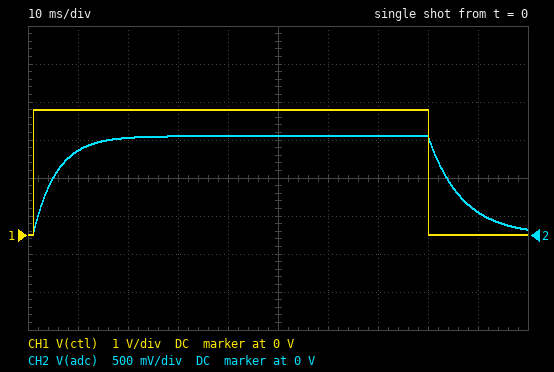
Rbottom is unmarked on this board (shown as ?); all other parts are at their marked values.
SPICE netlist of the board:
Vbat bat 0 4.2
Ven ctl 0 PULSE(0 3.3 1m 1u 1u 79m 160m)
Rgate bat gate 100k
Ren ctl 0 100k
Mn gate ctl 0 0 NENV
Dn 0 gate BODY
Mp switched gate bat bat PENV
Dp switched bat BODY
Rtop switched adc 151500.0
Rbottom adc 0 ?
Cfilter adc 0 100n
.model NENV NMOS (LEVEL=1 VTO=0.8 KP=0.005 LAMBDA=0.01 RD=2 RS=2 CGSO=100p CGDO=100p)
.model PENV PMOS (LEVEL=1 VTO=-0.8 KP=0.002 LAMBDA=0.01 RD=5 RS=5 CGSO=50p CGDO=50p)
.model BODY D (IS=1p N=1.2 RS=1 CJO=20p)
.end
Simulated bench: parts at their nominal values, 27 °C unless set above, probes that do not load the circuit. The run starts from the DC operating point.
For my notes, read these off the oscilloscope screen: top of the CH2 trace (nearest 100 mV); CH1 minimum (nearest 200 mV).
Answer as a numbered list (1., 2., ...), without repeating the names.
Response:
1. 1.3 V
2. 0 V
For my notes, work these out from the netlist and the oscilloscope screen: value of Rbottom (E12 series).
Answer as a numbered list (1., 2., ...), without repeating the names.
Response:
1. 68 kΩ
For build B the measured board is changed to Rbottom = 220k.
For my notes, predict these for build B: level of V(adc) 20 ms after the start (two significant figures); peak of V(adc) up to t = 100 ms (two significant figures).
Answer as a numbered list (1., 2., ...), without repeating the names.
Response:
1. 2.2 V
2. 2.5 V
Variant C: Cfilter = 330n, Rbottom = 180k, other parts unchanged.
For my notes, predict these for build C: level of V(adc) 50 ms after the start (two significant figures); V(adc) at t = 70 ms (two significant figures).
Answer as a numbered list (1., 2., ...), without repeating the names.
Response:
1. 1.9 V
2. 2.1 V
